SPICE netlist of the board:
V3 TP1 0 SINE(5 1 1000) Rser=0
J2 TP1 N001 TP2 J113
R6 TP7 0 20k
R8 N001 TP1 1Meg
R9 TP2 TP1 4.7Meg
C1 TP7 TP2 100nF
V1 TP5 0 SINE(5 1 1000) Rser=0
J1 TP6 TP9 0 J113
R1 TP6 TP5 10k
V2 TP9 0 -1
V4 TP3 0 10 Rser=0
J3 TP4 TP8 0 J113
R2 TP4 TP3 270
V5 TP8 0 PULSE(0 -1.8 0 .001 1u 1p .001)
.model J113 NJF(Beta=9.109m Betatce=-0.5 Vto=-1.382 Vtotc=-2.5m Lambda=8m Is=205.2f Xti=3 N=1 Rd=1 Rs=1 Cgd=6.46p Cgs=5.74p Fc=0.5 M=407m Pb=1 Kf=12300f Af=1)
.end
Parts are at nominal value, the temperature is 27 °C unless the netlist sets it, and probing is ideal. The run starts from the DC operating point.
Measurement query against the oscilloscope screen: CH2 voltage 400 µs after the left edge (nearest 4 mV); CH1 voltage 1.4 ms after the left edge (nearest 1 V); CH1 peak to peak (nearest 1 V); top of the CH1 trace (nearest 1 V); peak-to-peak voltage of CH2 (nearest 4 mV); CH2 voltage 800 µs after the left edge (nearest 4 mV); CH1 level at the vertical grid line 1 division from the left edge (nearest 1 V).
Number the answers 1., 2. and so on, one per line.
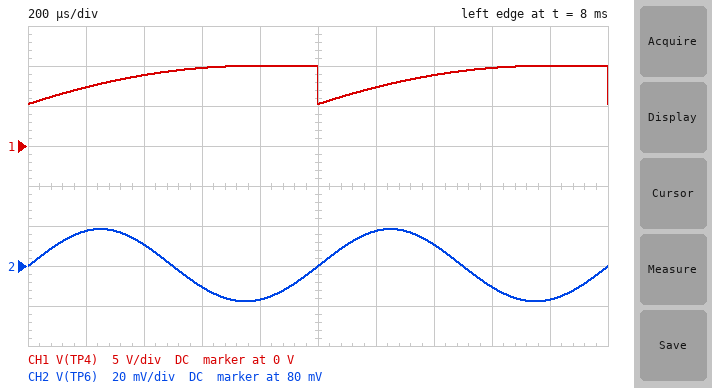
1. 92 mV
2. 9 V
3. 5 V
4. 10 V
5. 36 mV
6. 64 mV
7. 7 V
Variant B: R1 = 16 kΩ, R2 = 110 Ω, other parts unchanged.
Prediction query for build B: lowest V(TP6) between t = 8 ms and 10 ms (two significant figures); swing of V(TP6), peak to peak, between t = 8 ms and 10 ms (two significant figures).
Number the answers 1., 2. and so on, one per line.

1. 38 mV
2. 21 mV
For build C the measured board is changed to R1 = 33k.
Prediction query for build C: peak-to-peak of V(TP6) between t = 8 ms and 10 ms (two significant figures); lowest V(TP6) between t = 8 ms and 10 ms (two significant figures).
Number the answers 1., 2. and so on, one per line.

1. 9.3 mV
2. 18 mV
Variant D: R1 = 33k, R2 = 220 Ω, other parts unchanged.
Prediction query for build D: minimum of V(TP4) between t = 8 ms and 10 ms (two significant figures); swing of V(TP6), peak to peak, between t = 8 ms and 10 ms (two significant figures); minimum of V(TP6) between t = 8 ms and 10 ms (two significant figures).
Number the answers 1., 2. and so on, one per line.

1. 6.1 V
2. 9.3 mV
3. 18 mV
